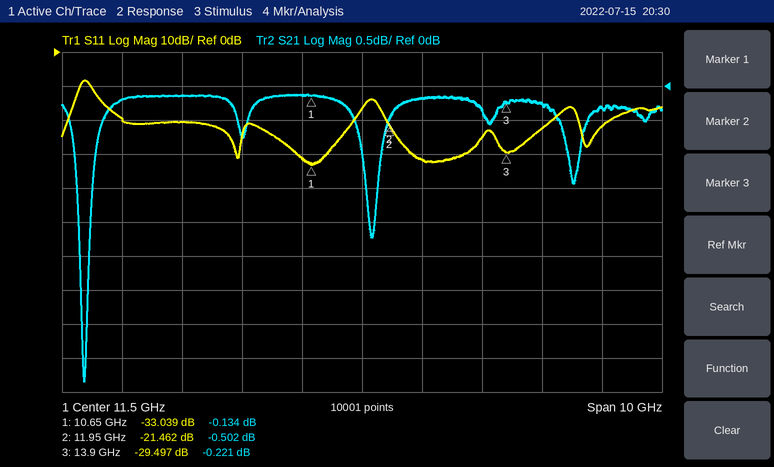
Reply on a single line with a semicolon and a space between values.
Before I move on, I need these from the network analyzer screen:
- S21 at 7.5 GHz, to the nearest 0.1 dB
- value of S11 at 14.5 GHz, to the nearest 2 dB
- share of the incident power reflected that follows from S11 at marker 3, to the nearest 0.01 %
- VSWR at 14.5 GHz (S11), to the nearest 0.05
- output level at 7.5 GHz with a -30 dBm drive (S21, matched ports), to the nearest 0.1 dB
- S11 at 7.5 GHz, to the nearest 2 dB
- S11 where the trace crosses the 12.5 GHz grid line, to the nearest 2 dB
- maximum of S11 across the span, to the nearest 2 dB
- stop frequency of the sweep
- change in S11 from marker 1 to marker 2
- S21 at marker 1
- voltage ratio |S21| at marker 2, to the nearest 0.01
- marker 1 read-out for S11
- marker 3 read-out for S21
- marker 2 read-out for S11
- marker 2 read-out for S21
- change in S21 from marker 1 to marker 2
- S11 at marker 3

-0.2 dB; -22 dB; 0.11 %; 1.15; -30.2 dBm; -20 dB; -32 dB; -8 dB; 16.5 GHz; 11.577 dB; -0.134 dB; 0.94; -33.039 dB; -0.221 dB; -21.462 dB; -0.502 dB; -0.368 dB; -29.497 dB
